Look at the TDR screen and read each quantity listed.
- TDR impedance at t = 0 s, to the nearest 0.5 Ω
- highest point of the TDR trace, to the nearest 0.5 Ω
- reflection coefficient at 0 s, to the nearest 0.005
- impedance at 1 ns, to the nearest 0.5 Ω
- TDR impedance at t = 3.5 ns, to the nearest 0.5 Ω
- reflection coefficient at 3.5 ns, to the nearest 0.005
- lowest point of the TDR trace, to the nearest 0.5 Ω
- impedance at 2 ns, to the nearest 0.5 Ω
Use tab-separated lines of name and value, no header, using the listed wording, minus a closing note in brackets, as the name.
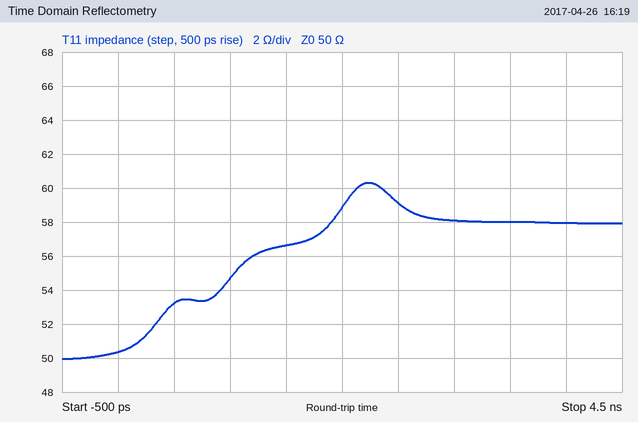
TDR impedance at t = 0 s, to the nearest 0.5 Ω	50.5 Ω
highest point of the TDR trace, to the nearest 0.5 Ω	60.5 Ω
reflection coefficient at 0 s, to the nearest 0.005	+0.005
impedance at 1 ns, to the nearest 0.5 Ω	54.5 Ω
TDR impedance at t = 3.5 ns, to the nearest 0.5 Ω	58.0 Ω
reflection coefficient at 3.5 ns, to the nearest 0.005	+0.075
lowest point of the TDR trace, to the nearest 0.5 Ω	50.0 Ω
impedance at 2 ns, to the nearest 0.5 Ω	59.0 Ω
